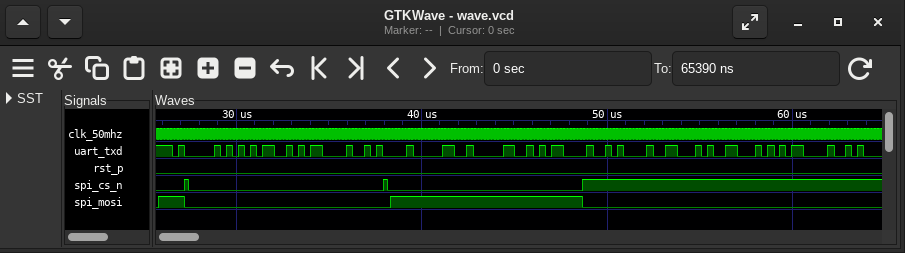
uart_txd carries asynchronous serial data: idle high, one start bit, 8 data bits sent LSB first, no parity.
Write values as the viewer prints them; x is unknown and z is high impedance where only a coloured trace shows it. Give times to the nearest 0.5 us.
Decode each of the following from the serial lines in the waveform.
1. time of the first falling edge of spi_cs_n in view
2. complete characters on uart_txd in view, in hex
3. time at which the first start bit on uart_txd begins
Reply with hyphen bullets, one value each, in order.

- 27.5 us
- 41, 35, 0D, 0A, 30, 30, 0D, 0A, 46, 46, 0D
- 26.5 us
